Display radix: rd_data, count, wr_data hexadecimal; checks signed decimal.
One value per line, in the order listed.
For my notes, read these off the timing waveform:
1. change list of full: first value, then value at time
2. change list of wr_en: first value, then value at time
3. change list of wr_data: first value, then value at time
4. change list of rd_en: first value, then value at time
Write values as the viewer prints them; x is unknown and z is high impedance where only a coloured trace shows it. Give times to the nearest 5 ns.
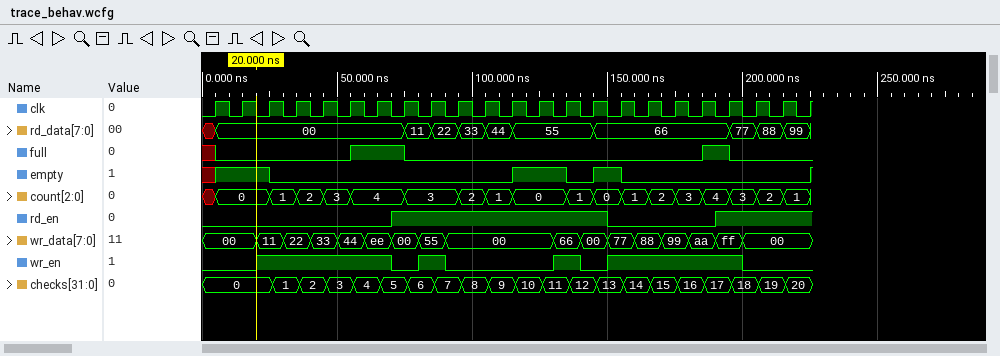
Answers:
x, 0 at 5 ns, 1 at 55 ns, 0 at 75 ns, 1 at 185 ns, 0 at 195 ns
0, 1 at 20 ns, 0 at 70 ns, 1 at 80 ns, 0 at 90 ns, 1 at 130 ns, 0 at 140 ns, 1 at 150 ns, 0 at 200 ns
00, 11 at 20 ns, 22 at 30 ns, 33 at 40 ns, 44 at 50 ns, ee at 60 ns, 00 at 70 ns, 55 at 80 ns, 00 at 90 ns, 66 at 130 ns, 00 at 140 ns, 77 at 150 ns, 88 at 160 ns, 99 at 170 ns, aa at 180 ns, ff at 190 ns, 00 at 200 ns
0, 1 at 70 ns, 0 at 150 ns, 1 at 190 ns
